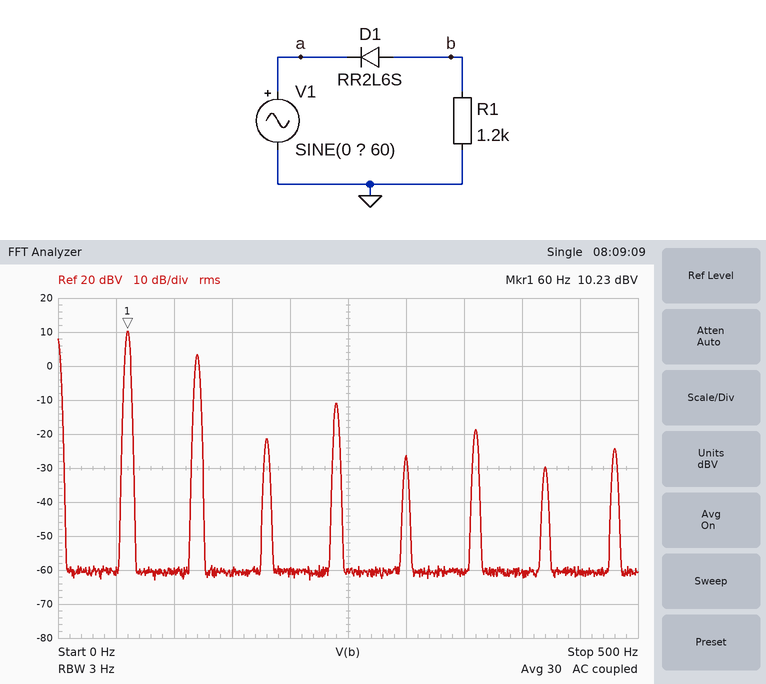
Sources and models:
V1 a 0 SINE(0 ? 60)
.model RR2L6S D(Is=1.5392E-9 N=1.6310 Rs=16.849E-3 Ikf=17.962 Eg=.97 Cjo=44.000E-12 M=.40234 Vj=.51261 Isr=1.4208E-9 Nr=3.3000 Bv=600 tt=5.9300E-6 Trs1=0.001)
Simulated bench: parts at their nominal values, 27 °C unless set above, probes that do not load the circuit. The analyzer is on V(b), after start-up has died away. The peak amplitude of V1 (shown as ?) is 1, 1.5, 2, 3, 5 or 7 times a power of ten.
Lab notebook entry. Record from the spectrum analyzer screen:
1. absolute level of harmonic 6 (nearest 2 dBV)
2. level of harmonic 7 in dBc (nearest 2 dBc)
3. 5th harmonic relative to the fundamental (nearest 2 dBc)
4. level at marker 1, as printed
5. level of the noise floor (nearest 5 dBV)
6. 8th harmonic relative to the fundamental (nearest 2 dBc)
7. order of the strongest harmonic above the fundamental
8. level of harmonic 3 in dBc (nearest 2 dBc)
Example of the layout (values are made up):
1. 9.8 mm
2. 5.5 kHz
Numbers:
1. -18 dBV
2. -40 dBc
3. -36 dBc
4. 10.23 dBV
5. -60 dBV
6. -34 dBc
7. 2
8. -32 dBc
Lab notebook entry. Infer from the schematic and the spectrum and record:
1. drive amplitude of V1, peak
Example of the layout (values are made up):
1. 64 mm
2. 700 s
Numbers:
1. 10 V
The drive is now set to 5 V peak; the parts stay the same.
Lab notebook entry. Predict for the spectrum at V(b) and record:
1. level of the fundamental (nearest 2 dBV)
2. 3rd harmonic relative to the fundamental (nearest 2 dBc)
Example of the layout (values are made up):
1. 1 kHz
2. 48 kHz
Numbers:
1. 4 dBV
2. -26 dBc
